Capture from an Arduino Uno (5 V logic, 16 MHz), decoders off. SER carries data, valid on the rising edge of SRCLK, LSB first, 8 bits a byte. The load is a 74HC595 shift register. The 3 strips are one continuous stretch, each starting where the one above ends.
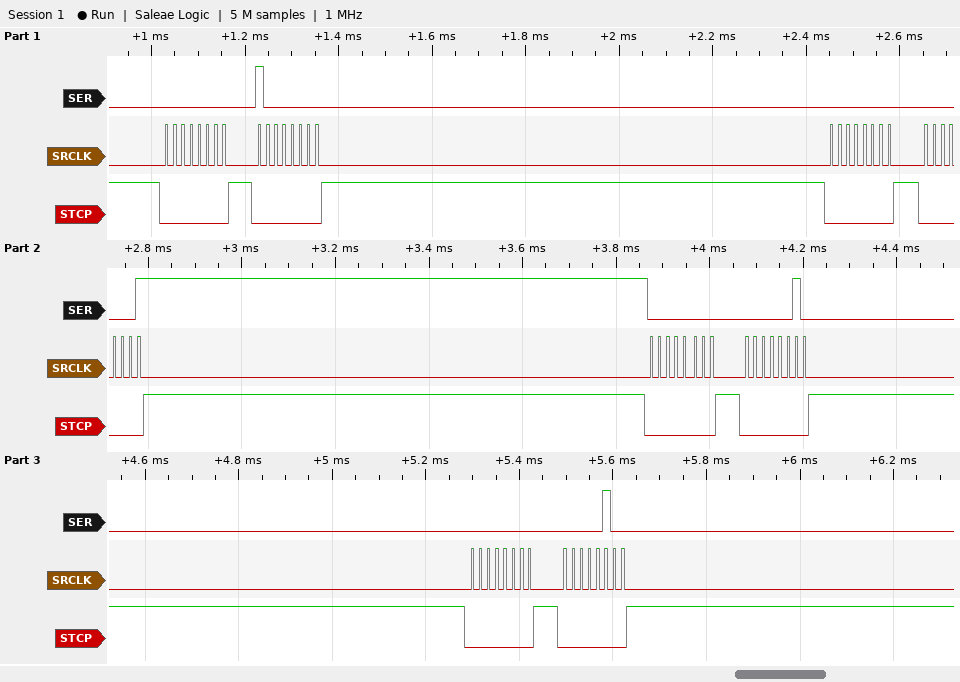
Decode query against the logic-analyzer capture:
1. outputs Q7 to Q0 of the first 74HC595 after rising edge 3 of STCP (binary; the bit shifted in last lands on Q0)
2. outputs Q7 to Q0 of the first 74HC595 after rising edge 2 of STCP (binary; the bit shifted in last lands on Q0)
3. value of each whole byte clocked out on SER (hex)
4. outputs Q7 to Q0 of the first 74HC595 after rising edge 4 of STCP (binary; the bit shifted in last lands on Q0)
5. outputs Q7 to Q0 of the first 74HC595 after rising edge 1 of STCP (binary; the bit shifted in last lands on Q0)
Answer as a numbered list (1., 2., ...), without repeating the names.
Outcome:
1. 00000000
2. 10000000
3. 00 01 00 80 00 40 00 20
4. 00000001
5. 00000000
